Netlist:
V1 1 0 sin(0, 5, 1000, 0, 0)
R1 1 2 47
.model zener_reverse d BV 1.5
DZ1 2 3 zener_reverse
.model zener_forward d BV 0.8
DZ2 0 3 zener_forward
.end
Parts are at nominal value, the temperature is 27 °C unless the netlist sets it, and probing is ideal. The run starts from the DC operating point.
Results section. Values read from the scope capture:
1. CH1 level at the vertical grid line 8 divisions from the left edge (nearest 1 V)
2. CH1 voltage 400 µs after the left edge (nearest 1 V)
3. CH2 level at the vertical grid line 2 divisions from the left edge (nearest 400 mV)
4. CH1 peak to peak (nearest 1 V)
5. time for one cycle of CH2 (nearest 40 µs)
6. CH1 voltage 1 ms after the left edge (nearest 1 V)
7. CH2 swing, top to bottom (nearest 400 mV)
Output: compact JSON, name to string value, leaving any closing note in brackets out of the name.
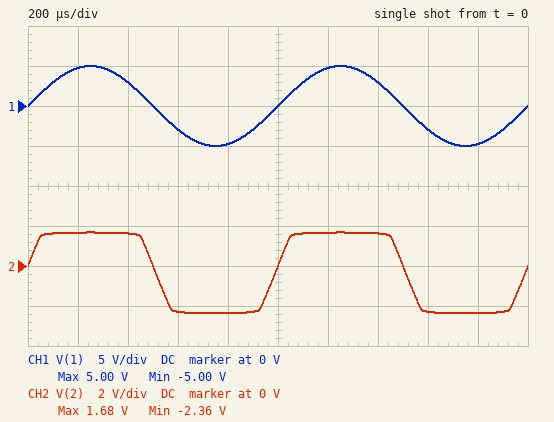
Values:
{"CH1 level at the vertical grid line 8 divisions from the left edge": "-3 V", "CH1 voltage 400 µs after the left edge": "3 V", "CH2 level at the vertical grid line 2 divisions from the left edge": "1.6 V", "CH1 peak to peak": "10 V", "time for one cycle of CH2": "1.00 ms", "CH1 voltage 1 ms after the left edge": "0 V", "CH2 swing, top to bottom": "4.0 V"}
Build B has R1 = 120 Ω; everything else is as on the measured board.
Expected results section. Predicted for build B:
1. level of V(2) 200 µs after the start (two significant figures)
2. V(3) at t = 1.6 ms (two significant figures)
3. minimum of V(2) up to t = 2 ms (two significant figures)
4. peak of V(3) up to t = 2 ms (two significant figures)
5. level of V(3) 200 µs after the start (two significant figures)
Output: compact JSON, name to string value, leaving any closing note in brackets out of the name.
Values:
{"level of V(2) 200 µs after the start": "1.6 V", "V(3) at t = 1.6 ms": "-700 mV", "minimum of V(2) up to t = 2 ms": "-2.3 V", "peak of V(3) up to t = 2 ms": "890 mV", "level of V(3) 200 µs after the start": "880 mV"}
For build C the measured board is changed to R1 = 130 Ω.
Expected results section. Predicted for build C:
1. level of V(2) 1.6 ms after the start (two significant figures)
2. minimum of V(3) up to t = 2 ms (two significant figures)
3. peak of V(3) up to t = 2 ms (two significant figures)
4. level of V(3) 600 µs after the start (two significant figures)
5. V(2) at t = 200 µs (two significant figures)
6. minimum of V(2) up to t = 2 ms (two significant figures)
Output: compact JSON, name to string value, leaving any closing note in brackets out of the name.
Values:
{"level of V(2) 1.6 ms after the start": "-2.2 V", "minimum of V(3) up to t = 2 ms": "-730 mV", "peak of V(3) up to t = 2 ms": "880 mV", "level of V(3) 600 µs after the start": "-700 mV", "V(2) at t = 200 µs": "1.6 V", "minimum of V(2) up to t = 2 ms": "-2.3 V"}
